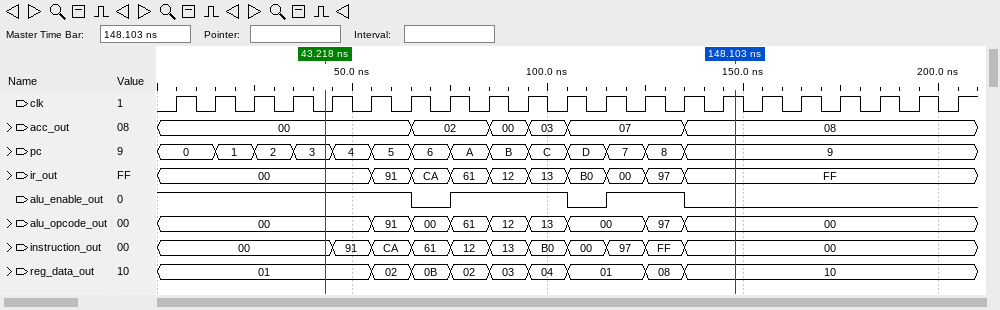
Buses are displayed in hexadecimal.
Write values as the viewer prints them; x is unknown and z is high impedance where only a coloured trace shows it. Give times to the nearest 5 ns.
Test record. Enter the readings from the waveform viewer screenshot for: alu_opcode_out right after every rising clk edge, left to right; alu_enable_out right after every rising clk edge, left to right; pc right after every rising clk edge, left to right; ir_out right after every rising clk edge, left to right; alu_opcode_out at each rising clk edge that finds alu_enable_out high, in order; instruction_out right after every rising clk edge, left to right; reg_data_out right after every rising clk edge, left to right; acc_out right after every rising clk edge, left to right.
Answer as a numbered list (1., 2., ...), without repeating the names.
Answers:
1. 00, 00, 00, 00, 00, 91, 00, 61, 12, 13, 00, 00, 97, 00, 00, 00, 00, 00, 00, 00, 00
2. 1 1 1 1 1 1 0 1 1 1 0 1 1 0 0 0 0 0 0 0 0
3. 0, 1, 2, 3, 4, 5, 6, A, B, C, D, 7, 8, 9, 9, 9, 9, 9, 9, 9, 9
4. 00, 00, 00, 00, 00, 91, CA, 61, 12, 13, B0, 00, 97, FF, FF, FF, FF, FF, FF, FF, FF
5. 00, 00, 00, 00, 00, 00, 91, 61, 12, 13, 00, 97
6. 00, 00, 00, 00, 91, CA, 61, 12, 13, B0, 00, 97, FF, 00, 00, 00, 00, 00, 00, 00, 00
7. 01, 01, 01, 01, 01, 02, 0B, 02, 03, 04, 01, 01, 08, 10, 10, 10, 10, 10, 10, 10, 10
8. 00, 00, 00, 00, 00, 00, 02, 02, 00, 03, 07, 07, 07, 08, 08, 08, 08, 08, 08, 08, 08
